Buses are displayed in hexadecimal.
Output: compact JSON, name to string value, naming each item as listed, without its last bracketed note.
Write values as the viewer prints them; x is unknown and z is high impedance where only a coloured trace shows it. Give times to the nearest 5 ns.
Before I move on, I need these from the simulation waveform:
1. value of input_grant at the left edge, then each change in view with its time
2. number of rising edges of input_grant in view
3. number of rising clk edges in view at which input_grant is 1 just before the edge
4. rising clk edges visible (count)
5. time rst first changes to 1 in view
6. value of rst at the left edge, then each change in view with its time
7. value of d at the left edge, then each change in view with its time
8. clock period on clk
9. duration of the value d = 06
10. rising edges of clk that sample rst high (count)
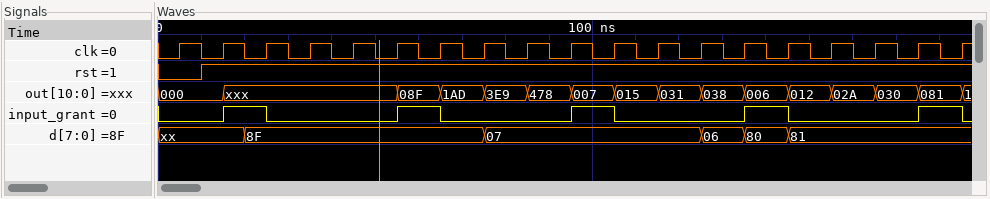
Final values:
{"value of input_grant at the left edge, then each change in view with its time": "0, 1 at 15 ns, 0 at 25 ns, 1 at 55 ns, 0 at 65 ns, 1 at 95 ns, 0 at 105 ns, 1 at 135 ns, 0 at 145 ns, 1 at 175 ns, 0 at 185 ns", "number of rising edges of input_grant in view": "5", "number of rising clk edges in view at which input_grant is 1 just before the edge": "5", "rising clk edges visible": "19", "time rst first changes to 1 in view": "10 ns", "value of rst at the left edge, then each change in view with its time": "0, 1 at 10 ns", "value of d at the left edge, then each change in view with its time": "xx, 8F at 20 ns, 07 at 75 ns, 06 at 125 ns, 80 at 135 ns, 81 at 145 ns", "clock period on clk": "10 ns", "duration of the value d = 06": "10 ns", "rising edges of clk that sample rst high": "18"}
